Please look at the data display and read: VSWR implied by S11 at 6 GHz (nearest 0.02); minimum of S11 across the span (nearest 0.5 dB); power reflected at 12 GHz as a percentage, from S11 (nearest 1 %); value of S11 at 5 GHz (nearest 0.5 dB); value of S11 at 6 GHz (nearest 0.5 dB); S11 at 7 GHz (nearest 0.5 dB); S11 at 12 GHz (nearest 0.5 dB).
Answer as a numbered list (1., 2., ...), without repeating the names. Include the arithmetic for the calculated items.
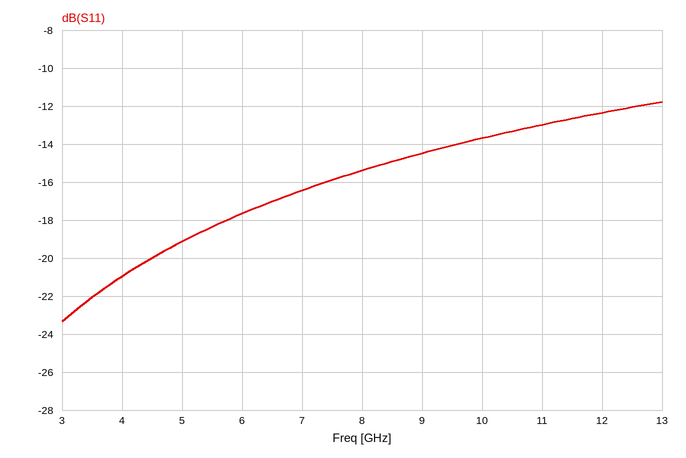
1. |Γ| = 10^(-17.5/20) = 0.1334; VSWR = (1 + 0.1334)/(1 − 0.1334) ≈ 1.31, so 1.30 to the nearest 0.02
2. -23.5 dB
3. 10^(-12.5/10) ≈ 6 %
4. -19.0 dB
5. -17.5 dB
6. -16.5 dB
7. -12.5 dB
